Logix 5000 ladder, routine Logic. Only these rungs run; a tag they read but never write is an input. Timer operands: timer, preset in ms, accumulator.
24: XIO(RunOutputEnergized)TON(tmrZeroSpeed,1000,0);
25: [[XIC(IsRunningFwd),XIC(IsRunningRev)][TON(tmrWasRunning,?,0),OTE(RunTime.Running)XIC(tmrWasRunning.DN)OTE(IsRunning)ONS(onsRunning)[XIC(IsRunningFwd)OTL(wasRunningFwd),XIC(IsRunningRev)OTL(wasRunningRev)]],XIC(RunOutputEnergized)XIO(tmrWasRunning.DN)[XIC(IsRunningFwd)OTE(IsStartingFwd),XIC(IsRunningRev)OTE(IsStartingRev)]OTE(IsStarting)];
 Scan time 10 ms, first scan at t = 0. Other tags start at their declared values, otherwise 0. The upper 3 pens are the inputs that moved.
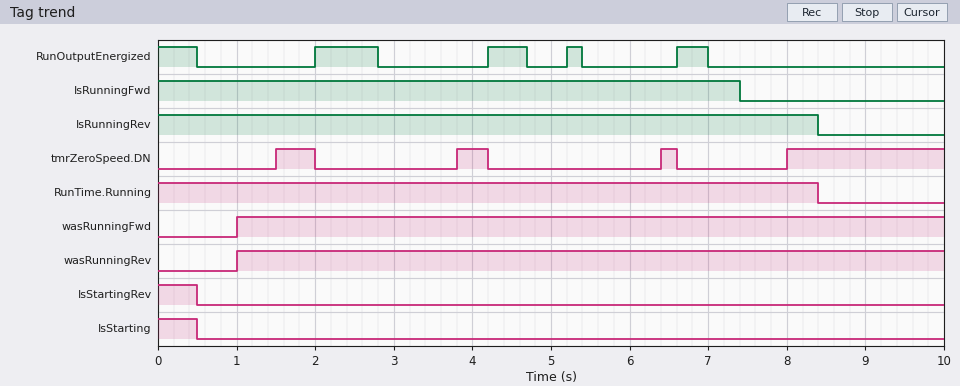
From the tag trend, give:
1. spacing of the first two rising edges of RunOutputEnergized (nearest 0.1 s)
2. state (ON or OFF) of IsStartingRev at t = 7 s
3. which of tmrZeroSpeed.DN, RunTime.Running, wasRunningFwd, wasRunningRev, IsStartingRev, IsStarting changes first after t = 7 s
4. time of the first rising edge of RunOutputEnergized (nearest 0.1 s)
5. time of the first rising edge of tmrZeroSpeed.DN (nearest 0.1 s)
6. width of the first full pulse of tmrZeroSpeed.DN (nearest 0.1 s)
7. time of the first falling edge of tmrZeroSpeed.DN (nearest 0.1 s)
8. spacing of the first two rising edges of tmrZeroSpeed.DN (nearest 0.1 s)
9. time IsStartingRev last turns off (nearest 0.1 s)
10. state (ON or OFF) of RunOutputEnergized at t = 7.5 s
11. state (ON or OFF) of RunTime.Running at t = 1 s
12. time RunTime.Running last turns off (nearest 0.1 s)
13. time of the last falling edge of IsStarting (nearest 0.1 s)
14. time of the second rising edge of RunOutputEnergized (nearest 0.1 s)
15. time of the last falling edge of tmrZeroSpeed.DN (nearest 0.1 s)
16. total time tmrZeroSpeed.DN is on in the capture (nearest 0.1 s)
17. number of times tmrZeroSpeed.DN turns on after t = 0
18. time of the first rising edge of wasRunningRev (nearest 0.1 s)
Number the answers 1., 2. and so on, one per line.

1. 2.2 s
2. OFF
3. tmrZeroSpeed.DN
4. 2.0 s
5. 1.5 s
6. 0.5 s
7. 2.0 s
8. 2.3 s
9. 0.5 s
10. OFF
11. ON
12. 8.4 s
13. 0.5 s
14. 4.2 s
15. 6.6 s
16. 3.1 s
17. 4
18. 1.0 s
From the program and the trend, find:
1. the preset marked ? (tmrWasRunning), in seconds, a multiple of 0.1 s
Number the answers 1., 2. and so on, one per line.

1. 1.0 s
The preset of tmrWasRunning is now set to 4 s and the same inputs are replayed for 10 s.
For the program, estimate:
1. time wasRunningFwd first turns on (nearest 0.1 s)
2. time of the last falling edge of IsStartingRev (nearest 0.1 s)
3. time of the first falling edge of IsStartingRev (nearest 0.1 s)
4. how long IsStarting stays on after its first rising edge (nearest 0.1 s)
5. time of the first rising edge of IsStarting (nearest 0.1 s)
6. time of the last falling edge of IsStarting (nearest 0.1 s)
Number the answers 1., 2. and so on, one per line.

1. 4.0 s
2. 2.8 s
3. 0.5 s
4. 0.8 s
5. 2.0 s
6. 2.8 s
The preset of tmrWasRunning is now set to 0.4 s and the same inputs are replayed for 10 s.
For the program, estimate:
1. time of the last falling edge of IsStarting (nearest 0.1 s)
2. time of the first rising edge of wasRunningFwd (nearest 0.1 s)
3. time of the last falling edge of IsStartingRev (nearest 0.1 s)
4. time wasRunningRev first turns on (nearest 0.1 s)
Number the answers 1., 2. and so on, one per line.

1. 0.4 s
2. 0.4 s
3. 0.4 s
4. 0.4 s
